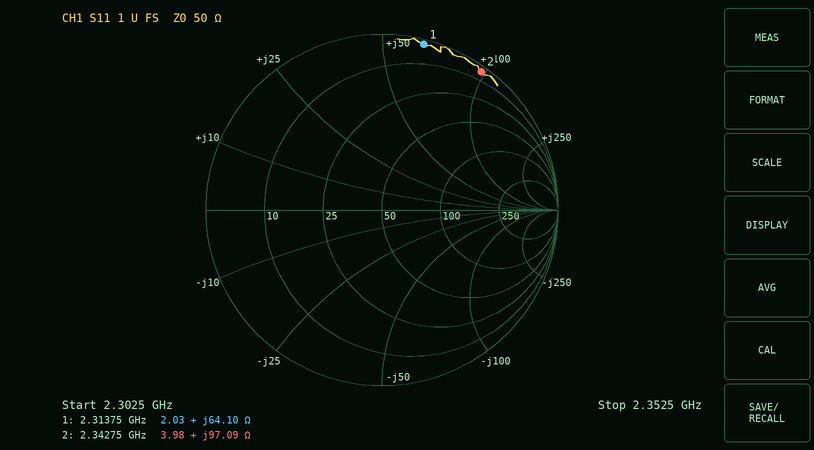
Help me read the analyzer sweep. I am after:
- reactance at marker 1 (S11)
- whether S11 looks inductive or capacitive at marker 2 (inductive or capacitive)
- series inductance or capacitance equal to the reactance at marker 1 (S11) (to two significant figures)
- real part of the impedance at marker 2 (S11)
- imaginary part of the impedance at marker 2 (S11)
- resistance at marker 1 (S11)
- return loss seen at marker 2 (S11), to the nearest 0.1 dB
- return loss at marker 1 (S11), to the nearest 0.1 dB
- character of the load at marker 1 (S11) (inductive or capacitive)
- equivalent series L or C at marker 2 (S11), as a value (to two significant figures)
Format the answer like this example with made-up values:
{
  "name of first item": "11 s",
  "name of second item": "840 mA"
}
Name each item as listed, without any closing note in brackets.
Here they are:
{
  "reactance at marker 1": "+64.10 Ω",
  "whether S11 looks inductive or capacitive at marker 2": "inductive",
  "series inductance or capacitance equal to the reactance at marker 1 (S11)": "4.4 nH",
  "real part of the impedance at marker 2": "3.98 Ω",
  "imaginary part of the impedance at marker 2": "+97.09 Ω",
  "resistance at marker 1": "2.03 Ω",
  "return loss seen at marker 2 (S11), to the nearest 0.1 dB": "0.3 dB",
  "return loss at marker 1 (S11), to the nearest 0.1 dB": "0.3 dB",
  "character of the load at marker 1 (S11)": "inductive",
  "equivalent series L or C at marker 2 (S11), as a value": "6.6 nH"
}
